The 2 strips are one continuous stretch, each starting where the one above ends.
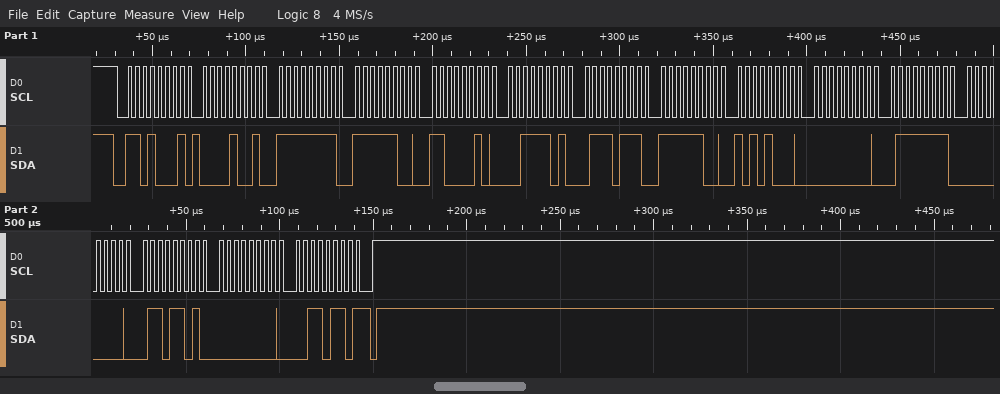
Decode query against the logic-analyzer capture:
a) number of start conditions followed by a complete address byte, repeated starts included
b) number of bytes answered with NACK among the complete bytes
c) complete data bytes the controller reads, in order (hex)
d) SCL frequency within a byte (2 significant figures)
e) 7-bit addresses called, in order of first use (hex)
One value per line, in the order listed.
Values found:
1
1
09 FF FC C2 3D 77 FC A8 00 7F 00 6D 00 36
250 kHz
0x68
